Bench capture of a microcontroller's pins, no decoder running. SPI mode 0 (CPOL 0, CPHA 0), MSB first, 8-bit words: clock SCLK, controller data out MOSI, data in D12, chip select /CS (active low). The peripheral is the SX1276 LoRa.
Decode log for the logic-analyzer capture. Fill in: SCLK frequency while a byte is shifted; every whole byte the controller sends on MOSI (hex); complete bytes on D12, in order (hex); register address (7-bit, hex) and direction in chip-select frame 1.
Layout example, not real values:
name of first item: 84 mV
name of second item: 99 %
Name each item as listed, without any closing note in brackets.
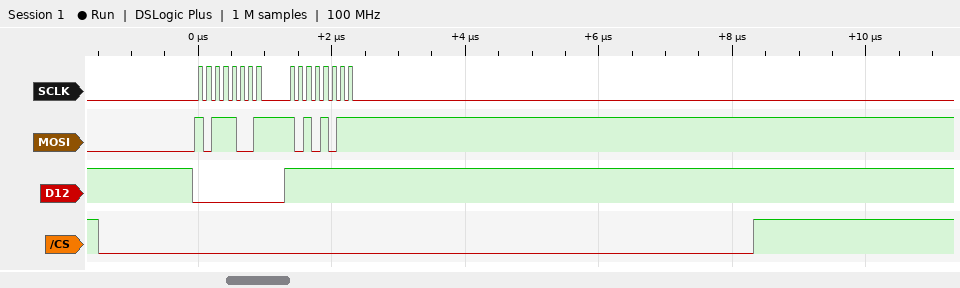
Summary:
SCLK frequency while a byte is shifted: 8 MHz
every whole byte the controller sends on MOSI: 0xB9 0xAB
complete bytes on D12, in order: 0x00 0xFF
register address (7-bit, hex) and direction in chip-select frame 1: 0x39 write
